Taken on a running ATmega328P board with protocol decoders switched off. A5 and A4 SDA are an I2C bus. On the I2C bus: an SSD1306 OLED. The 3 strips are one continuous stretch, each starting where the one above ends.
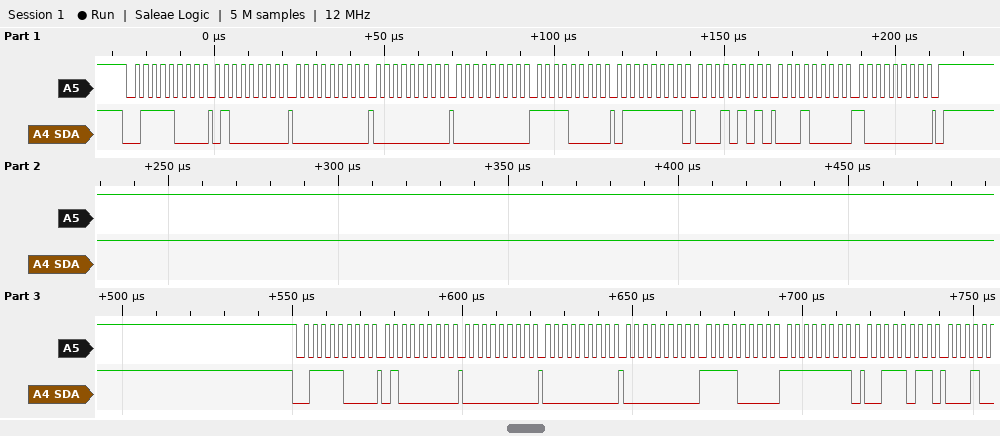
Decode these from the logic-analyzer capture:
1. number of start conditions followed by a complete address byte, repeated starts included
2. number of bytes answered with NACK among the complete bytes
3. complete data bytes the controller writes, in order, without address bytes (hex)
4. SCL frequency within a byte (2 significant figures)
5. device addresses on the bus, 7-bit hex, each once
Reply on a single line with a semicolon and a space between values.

2; 0; 40 00 00 00 F0 7F 15 10 80 40 00 00 00 F0 FF 3B; 400 kHz; 0x3C
